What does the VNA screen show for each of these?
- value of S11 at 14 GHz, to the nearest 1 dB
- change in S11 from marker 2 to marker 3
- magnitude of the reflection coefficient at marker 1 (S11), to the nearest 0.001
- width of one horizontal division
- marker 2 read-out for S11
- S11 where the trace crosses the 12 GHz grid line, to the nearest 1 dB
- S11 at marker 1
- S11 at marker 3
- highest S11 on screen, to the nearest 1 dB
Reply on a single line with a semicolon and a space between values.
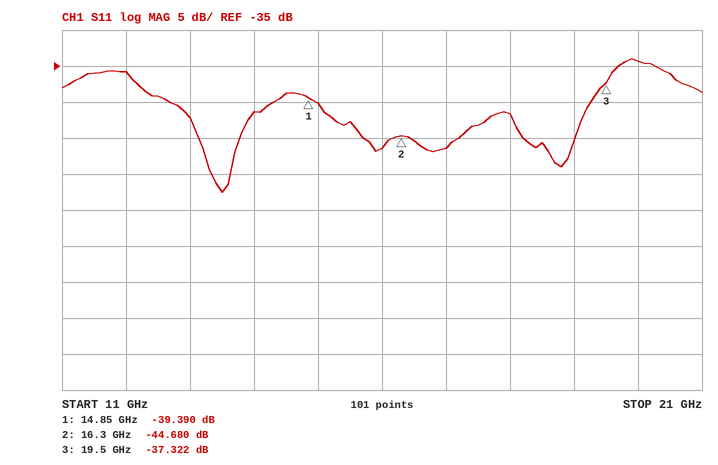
-41 dB; 7.358 dB; 0.011; 1 GHz; -44.680 dB; -36 dB; -39.390 dB; -37.322 dB; -34 dB
